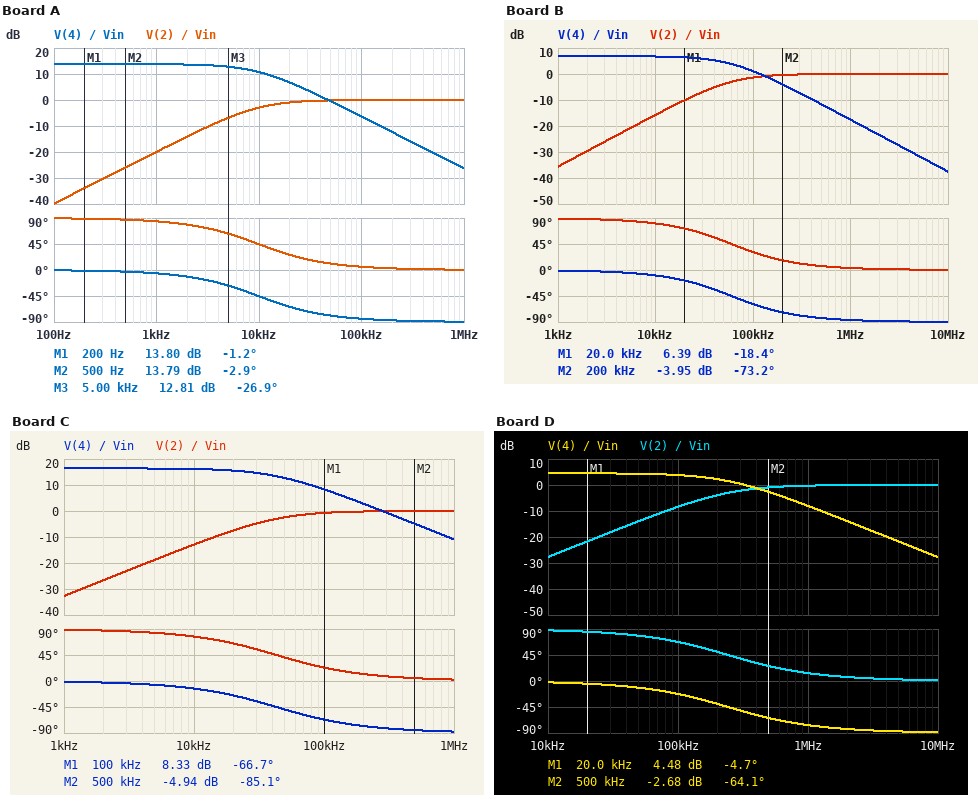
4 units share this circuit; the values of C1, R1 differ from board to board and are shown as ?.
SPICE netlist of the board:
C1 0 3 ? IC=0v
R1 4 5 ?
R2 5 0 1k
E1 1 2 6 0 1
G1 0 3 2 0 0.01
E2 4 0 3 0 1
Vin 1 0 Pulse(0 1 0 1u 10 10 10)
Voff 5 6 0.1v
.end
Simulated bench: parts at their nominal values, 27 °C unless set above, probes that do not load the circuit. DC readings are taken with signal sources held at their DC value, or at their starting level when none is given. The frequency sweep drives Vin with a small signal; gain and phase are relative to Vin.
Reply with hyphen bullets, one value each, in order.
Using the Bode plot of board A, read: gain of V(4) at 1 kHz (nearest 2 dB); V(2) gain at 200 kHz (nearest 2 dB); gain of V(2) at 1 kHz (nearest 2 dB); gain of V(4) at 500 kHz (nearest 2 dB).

- 14 dB
- 0 dB
- -20 dB
- -20 dB
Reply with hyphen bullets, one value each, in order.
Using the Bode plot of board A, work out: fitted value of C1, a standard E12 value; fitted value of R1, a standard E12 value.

- 33 nF
- 3.9 kΩ
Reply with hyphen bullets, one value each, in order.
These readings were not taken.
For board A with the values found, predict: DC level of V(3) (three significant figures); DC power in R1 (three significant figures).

- 490 mV
- 39.0 µW
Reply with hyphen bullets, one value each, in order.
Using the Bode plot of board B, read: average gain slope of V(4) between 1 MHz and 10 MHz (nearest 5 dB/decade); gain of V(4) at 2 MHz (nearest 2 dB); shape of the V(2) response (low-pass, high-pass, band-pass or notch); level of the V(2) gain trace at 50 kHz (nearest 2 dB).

- -20 dB/decade
- -24 dB
- high-pass
- -4 dB
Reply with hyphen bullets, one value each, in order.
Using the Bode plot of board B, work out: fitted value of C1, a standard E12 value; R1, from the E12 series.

- 12 nF
- 1.2 kΩ
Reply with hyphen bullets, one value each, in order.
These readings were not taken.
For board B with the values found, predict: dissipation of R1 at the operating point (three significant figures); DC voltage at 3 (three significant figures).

- 12.0 µW
- 220 mV
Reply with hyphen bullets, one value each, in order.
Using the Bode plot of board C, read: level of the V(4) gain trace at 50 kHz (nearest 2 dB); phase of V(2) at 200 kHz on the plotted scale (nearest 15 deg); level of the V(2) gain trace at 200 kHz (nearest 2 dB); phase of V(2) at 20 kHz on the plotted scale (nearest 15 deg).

- 12 dB
- 15 deg
- 0 dB
- 60 deg
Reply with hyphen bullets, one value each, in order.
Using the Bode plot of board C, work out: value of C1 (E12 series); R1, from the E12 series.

- 5.6 nF
- 5.6 kΩ
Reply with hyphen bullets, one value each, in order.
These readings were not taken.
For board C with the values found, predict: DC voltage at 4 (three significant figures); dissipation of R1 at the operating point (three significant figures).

- 660 mV
- 56.0 µW
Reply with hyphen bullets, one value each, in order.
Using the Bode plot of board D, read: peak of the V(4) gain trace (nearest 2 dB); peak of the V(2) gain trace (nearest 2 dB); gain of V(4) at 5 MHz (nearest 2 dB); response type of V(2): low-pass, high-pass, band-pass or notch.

- 4 dB
- 0 dB
- -22 dB
- high-pass
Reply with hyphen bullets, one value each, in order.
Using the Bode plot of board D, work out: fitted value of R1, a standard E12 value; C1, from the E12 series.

- 680 Ω
- 3.9 nF
